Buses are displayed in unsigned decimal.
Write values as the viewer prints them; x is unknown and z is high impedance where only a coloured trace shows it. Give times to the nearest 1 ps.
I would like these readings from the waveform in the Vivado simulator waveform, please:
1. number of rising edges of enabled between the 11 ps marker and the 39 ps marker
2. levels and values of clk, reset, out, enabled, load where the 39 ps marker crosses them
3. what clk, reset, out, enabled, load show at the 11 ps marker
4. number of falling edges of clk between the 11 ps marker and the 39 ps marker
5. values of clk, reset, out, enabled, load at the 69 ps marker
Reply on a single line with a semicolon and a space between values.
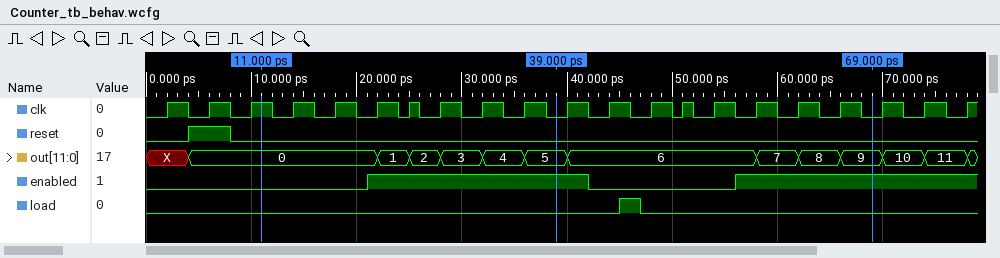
1; clk=0, reset=0, out=5, enabled=1, load=0; clk=1, reset=0, out=0, enabled=0, load=0; 8; clk=0, reset=0, out=9, enabled=1, load=0
